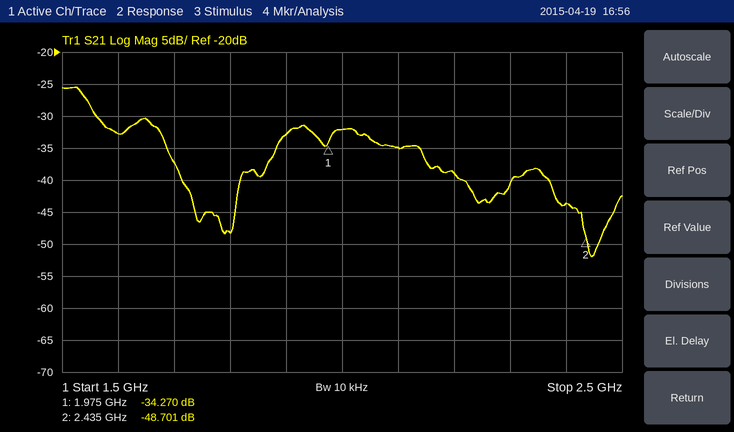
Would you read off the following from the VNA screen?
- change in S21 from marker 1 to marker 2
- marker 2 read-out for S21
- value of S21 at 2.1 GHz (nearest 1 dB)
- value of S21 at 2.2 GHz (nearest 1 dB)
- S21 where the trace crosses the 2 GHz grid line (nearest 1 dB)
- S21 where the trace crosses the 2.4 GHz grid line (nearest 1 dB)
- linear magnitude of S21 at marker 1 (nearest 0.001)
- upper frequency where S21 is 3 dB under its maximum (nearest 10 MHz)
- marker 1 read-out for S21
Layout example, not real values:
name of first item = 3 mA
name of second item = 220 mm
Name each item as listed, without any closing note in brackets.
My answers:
change in S21 from marker 1 to marker 2 = -14.431 dB
marker 2 read-out for S21 = -48.701 dB
value of S21 at 2.1 GHz = -35 dB
value of S21 at 2.2 GHz = -39 dB
S21 where the trace crosses the 2 GHz grid line = -32 dB
S21 where the trace crosses the 2.4 GHz grid line = -44 dB
linear magnitude of S21 at marker 1 = 0.019
upper frequency where S21 is 3 dB under its maximum = 1.55 GHz
marker 1 read-out for S21 = -34.270 dB
